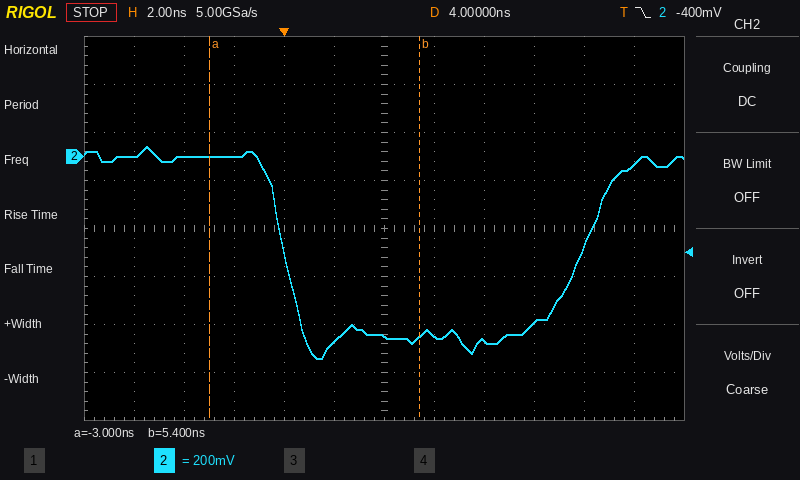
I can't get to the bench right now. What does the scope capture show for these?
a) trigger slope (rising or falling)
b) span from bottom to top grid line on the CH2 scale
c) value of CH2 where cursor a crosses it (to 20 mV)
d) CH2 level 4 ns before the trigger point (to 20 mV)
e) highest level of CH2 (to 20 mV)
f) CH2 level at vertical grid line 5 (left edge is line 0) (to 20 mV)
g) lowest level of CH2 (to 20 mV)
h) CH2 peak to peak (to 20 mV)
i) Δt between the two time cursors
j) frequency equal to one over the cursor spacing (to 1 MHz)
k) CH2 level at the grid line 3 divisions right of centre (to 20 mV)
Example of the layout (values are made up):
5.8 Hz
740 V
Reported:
falling
1.6 V
0 mV
0 mV
40 mV
-780 mV
-840 mV
880 mV
8.4 ns
119 MHz
-700 mV
